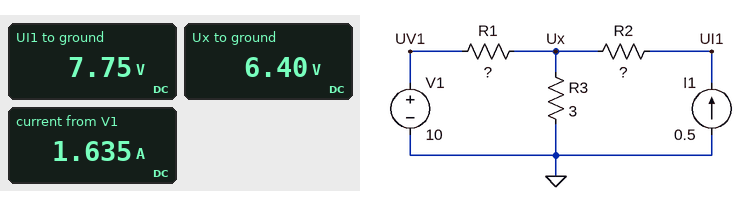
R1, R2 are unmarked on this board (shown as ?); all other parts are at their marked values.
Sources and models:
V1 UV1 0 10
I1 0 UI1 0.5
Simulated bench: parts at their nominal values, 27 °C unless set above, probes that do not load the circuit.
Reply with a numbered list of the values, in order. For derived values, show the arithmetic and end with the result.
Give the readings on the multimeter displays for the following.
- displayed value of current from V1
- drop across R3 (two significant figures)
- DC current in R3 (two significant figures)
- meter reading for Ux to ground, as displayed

1. 1.635 A
2. 6.4 V = 6.4 V
3. (6.4 V) / 3 Ω = 2.1 A
4. 6.40 V
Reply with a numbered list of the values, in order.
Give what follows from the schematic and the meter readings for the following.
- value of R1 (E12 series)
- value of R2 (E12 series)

1. 2.2 Ω
2. 2.7 Ω
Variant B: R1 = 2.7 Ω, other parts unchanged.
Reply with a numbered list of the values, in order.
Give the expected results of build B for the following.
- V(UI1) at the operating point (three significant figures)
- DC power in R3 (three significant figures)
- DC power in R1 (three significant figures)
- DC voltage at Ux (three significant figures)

1. 7.32 V
2. 11.9 W
3. 6.00 W
4. 5.97 V
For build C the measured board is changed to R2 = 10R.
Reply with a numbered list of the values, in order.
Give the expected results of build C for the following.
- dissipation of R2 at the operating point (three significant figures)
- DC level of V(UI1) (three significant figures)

1. 2.50 W
2. 11.4 V
